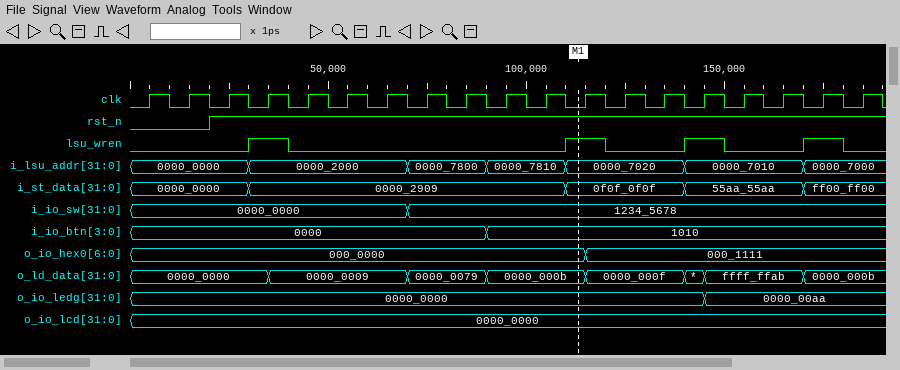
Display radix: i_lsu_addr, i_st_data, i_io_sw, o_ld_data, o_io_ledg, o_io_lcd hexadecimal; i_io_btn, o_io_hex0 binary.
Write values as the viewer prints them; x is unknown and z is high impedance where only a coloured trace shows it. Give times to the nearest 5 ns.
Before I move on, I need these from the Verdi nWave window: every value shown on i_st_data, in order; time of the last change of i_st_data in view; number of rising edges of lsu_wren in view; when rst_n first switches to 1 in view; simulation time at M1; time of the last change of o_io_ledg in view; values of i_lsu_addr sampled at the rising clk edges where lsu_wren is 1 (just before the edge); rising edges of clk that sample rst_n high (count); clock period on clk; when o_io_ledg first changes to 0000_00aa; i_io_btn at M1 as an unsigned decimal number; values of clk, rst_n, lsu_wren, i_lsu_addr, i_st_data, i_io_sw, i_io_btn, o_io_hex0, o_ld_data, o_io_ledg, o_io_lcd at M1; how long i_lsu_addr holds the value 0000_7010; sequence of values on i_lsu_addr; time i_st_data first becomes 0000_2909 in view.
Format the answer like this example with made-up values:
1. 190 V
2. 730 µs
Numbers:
1. 0000_0000, 0000_2909, 0f0f_0f0f, 55aa_55aa, ff00_ff00
2. 170 ns
3. 4
4. 20 ns
5. 115 ns
6. 145 ns
7. 0000_2000, 0000_7020, 0000_7010, 0000_7000
8. 17
9. 10 ns
10. 145 ns
11. 10
12. clk=0, rst_n=1, lsu_wren=1, i_lsu_addr=0000_7020, i_st_data=0f0f_0f0f, i_io_sw=1234_5678, i_io_btn=1010, o_io_hex0=000_0000, o_ld_data=0000_000b, o_io_ledg=0000_0000, o_io_lcd=0000_0000
13. 30 ns
14. 0000_0000, 0000_2000, 0000_7800, 0000_7810, 0000_7020, 0000_7010, 0000_7000
15. 30 ns
